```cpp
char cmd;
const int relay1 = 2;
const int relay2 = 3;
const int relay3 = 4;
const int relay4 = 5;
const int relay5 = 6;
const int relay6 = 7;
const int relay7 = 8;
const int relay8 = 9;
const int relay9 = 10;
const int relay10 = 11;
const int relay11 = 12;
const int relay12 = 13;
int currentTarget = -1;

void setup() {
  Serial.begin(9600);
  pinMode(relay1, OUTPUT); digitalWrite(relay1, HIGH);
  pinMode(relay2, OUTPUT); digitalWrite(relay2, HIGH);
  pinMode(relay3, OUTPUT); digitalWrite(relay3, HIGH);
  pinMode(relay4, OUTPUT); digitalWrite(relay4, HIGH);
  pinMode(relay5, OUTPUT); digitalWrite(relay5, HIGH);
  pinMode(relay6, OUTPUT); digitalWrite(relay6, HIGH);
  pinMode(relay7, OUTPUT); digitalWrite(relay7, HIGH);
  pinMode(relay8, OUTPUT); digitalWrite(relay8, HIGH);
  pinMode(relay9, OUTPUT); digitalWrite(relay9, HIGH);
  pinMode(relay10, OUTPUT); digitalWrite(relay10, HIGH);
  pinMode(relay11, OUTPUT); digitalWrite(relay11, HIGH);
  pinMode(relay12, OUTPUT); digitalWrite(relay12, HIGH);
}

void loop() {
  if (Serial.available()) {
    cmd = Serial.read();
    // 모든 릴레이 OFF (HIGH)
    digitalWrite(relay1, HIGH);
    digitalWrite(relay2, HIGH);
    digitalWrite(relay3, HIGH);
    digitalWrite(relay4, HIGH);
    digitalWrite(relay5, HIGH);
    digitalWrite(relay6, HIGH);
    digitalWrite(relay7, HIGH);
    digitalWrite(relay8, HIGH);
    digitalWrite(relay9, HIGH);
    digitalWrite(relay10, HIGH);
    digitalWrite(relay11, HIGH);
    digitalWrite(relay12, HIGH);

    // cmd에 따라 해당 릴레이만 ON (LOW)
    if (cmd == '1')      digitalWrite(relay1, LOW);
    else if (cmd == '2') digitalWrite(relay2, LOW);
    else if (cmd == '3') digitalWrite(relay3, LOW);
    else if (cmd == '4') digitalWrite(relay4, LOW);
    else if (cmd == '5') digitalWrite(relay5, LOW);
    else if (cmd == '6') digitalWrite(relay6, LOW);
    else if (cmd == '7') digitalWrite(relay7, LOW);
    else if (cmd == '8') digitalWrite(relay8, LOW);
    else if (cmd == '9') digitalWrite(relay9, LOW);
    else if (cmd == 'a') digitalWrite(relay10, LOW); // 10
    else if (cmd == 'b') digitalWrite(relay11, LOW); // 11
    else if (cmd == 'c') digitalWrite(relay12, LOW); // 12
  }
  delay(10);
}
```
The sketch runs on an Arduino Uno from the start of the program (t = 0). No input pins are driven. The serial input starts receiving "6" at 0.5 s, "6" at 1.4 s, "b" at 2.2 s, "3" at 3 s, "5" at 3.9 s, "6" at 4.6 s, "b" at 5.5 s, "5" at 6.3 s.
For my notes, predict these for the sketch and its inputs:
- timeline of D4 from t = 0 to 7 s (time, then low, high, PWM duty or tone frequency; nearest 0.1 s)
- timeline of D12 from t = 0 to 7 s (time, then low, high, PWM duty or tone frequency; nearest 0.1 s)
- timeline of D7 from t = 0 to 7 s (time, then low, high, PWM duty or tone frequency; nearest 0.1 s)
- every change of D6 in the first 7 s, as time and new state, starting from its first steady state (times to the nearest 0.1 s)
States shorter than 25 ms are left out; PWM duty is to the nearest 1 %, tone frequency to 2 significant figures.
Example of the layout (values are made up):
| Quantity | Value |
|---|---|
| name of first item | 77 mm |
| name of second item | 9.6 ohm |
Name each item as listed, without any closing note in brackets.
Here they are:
| Quantity | Value |
|---|---|
| timeline of D4 from t = 0 to 7 s | 0 s high; 3 s low; 3.9 s high |
| timeline of D12 from t = 0 to 7 s | 0 s high; 2.2 s low; 3 s high; 5.5 s low; 6.3 s high |
| timeline of D7 from t = 0 to 7 s | 0 s high; 0.5 s low; 2.2 s high; 4.6 s low; 5.5 s high |
| every change of D6 in the first 7 s, as time and new state, starting from its first steady state | 0 s high; 3.9 s low; 4.6 s high; 6.3 s low |
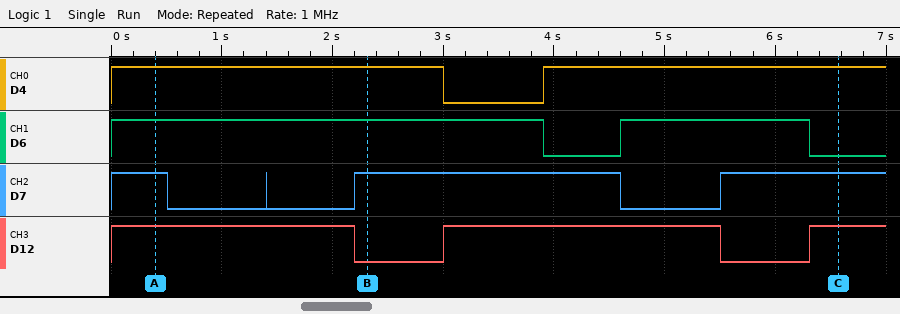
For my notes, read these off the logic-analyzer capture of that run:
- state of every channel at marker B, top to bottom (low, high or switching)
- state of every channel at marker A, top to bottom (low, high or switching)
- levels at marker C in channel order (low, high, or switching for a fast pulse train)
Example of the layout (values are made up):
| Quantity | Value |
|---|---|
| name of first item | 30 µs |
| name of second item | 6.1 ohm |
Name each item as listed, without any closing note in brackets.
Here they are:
| Quantity | Value |
|---|---|
| state of every channel at marker B, top to bottom | D4 high, D6 high, D7 high, D12 low |
| state of every channel at marker A, top to bottom | D4 high, D6 high, D7 high, D12 high |
| levels at marker C in channel order | D4 high, D6 low, D7 high, D12 high |
